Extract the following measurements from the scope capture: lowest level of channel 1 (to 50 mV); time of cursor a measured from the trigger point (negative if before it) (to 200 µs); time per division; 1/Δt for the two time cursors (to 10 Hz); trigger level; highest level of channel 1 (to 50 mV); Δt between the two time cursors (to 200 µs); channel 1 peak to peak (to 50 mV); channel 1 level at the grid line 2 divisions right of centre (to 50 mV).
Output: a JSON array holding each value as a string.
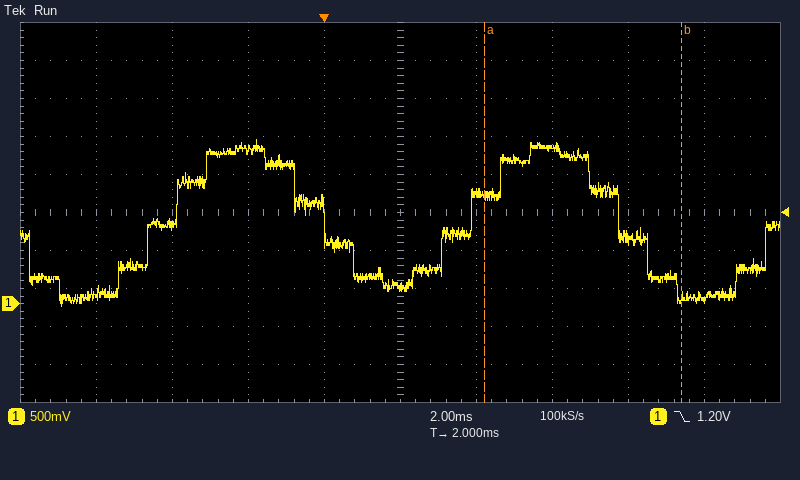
["-50 mV", "+4.2 ms", "2 ms", "190 Hz", "1.20 V", "2.15 V", "5.2 ms", "2.20 V", "2.05 V"]
